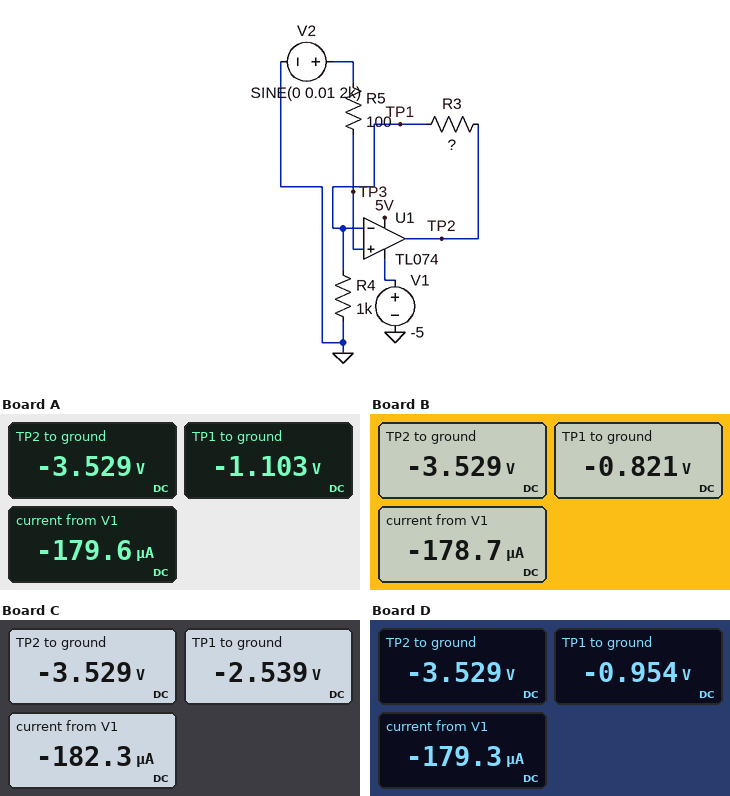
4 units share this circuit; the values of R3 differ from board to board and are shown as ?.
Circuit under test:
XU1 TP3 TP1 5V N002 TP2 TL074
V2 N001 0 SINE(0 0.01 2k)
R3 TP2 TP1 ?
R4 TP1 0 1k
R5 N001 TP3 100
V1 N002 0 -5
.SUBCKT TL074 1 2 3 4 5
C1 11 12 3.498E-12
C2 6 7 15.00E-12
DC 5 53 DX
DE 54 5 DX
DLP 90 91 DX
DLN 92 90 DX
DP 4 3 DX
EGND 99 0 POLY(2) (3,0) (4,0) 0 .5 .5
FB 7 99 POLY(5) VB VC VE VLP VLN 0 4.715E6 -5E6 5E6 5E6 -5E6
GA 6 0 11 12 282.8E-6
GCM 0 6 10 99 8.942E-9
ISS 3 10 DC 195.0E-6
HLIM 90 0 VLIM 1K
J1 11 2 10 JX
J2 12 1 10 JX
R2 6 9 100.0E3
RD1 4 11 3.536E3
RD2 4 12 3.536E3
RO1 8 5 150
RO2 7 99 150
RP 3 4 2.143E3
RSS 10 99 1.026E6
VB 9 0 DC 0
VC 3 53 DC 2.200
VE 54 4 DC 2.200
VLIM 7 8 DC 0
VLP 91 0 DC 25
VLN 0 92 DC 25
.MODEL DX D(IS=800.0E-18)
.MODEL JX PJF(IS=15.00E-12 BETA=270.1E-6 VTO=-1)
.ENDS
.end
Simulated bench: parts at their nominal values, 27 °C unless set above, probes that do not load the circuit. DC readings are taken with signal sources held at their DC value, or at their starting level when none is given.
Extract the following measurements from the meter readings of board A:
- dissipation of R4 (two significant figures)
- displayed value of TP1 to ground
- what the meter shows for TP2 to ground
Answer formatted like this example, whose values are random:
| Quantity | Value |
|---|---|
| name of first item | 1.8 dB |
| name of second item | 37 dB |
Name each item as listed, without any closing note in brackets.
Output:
| Quantity | Value |
|---|---|
| dissipation of R4 | 1.2 mW |
| displayed value of TP1 to ground | -1.103 V |
| what the meter shows for TP2 to ground | -3.529 V |
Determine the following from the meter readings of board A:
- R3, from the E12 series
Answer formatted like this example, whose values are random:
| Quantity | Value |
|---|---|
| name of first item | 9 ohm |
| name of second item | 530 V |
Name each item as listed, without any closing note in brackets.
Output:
| Quantity | Value |
|---|---|
| R3, from the E12 series | 2.2 kΩ |
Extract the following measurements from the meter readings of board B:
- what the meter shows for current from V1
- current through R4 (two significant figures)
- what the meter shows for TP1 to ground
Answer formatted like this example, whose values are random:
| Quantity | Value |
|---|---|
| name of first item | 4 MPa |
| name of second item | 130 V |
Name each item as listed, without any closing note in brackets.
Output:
| Quantity | Value |
|---|---|
| what the meter shows for current from V1 | -178.7 µA |
| current through R4 | 820 µA |
| what the meter shows for TP1 to ground | -0.821 V |
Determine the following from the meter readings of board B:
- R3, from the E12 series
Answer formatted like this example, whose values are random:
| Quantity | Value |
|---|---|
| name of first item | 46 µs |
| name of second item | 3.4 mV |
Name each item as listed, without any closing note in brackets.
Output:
| Quantity | Value |
|---|---|
| R3, from the E12 series | 3.3 kΩ |
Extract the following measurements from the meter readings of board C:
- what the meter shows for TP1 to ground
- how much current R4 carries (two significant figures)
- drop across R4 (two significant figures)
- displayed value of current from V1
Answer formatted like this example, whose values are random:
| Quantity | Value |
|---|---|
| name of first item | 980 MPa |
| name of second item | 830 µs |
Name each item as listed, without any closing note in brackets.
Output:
| Quantity | Value |
|---|---|
| what the meter shows for TP1 to ground | -2.539 V |
| how much current R4 carries | 2.5 mA |
| drop across R4 | 2.5 V |
| displayed value of current from V1 | -182.3 µA |
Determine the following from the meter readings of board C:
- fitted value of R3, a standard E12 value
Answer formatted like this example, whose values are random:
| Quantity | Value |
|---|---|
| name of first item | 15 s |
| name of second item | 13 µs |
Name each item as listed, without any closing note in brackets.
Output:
| Quantity | Value |
|---|---|
| fitted value of R3, a standard E12 value | 390 Ω |
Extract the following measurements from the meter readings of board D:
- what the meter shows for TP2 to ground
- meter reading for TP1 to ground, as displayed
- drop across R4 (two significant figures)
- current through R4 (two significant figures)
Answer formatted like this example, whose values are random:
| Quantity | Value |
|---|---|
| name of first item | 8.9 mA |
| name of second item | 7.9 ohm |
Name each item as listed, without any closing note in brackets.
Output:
| Quantity | Value |
|---|---|
| what the meter shows for TP2 to ground | -3.529 V |
| meter reading for TP1 to ground, as displayed | -0.954 V |
| drop across R4 | 950 mV |
| current through R4 | 950 µA |
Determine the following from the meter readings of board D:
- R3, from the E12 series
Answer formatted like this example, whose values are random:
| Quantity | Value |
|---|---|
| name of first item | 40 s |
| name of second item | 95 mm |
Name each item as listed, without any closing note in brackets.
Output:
| Quantity | Value |
|---|---|
| R3, from the E12 series | 2.7 kΩ |
